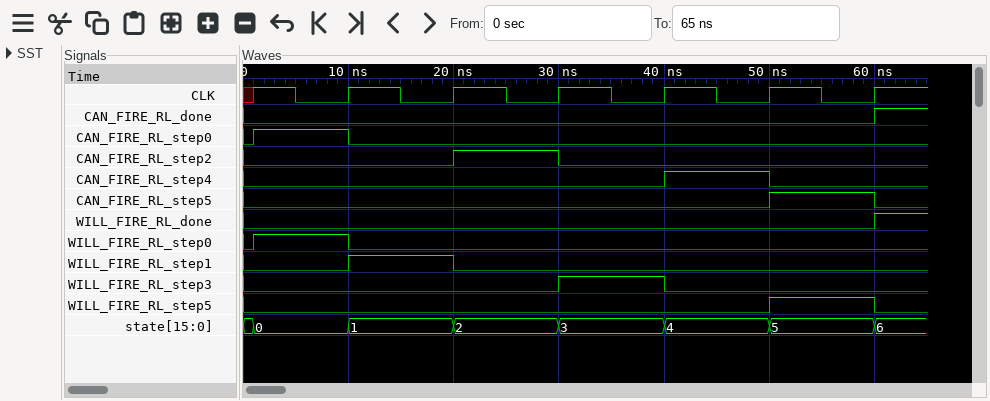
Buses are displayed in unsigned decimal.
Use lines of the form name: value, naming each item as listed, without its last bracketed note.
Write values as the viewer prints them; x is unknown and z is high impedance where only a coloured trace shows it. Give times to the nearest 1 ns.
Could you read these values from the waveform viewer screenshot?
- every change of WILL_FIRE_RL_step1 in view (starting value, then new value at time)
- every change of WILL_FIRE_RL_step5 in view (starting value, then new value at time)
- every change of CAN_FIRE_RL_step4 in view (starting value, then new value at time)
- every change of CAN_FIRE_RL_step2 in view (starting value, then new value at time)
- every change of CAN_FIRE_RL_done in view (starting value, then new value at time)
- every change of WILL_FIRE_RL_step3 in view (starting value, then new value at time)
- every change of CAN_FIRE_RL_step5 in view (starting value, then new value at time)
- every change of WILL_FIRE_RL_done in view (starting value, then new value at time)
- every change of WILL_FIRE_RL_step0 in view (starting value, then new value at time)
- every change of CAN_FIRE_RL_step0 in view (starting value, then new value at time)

every change of WILL_FIRE_RL_step1 in view: 0, 1 at 10 ns, 0 at 20 ns
every change of WILL_FIRE_RL_step5 in view: 0, 1 at 50 ns, 0 at 60 ns
every change of CAN_FIRE_RL_step4 in view: 0, 1 at 40 ns, 0 at 50 ns
every change of CAN_FIRE_RL_step2 in view: 0, 1 at 20 ns, 0 at 30 ns
every change of CAN_FIRE_RL_done in view: 0, 1 at 60 ns
every change of WILL_FIRE_RL_step3 in view: 0, 1 at 30 ns, 0 at 40 ns
every change of CAN_FIRE_RL_step5 in view: 0, 1 at 50 ns, 0 at 60 ns
every change of WILL_FIRE_RL_done in view: 0, 1 at 60 ns
every change of WILL_FIRE_RL_step0 in view: 0, 1 at 1 ns, 0 at 10 ns
every change of CAN_FIRE_RL_step0 in view: 0, 1 at 1 ns, 0 at 10 ns
